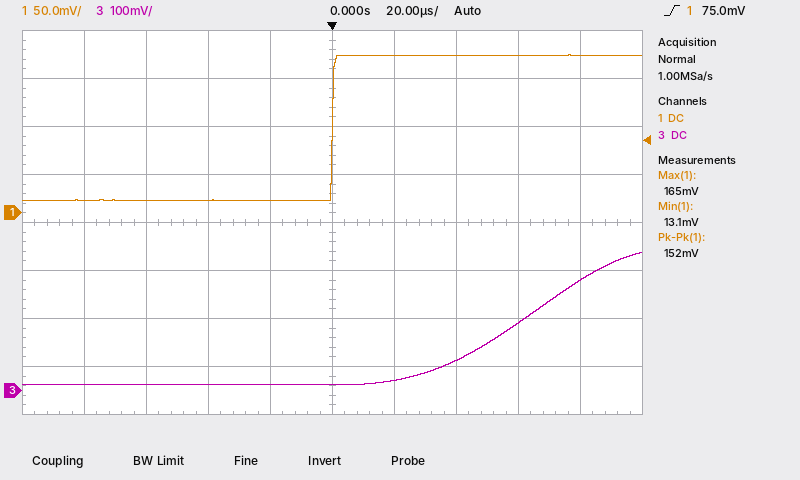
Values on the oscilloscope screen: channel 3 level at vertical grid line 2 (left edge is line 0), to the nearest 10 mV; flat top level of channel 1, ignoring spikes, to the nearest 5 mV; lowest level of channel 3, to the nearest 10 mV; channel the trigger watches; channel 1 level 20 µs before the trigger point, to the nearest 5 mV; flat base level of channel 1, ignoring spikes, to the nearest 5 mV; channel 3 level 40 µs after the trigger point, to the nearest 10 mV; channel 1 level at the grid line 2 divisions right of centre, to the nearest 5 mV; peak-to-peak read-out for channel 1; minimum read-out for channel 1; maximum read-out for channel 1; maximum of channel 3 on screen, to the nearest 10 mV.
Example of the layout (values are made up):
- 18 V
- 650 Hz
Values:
- 10 mV
- 165 mV
- 10 mV
- channel 1
- 15 mV
- 15 mV
- 60 mV
- 165 mV
- 152 mV
- 13.1 mV
- 165 mV
- 290 mV
